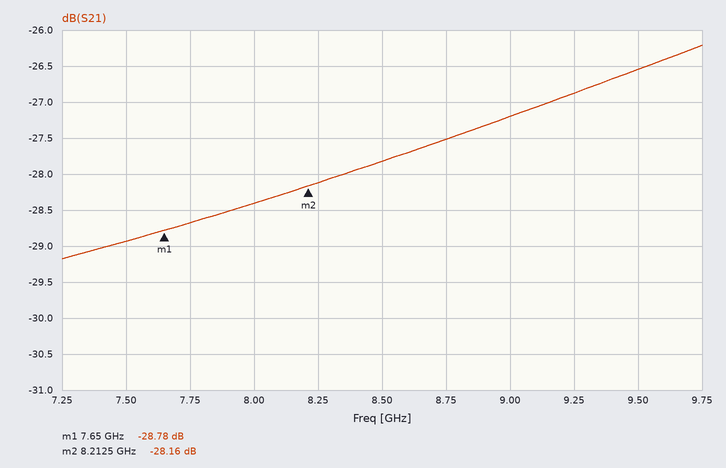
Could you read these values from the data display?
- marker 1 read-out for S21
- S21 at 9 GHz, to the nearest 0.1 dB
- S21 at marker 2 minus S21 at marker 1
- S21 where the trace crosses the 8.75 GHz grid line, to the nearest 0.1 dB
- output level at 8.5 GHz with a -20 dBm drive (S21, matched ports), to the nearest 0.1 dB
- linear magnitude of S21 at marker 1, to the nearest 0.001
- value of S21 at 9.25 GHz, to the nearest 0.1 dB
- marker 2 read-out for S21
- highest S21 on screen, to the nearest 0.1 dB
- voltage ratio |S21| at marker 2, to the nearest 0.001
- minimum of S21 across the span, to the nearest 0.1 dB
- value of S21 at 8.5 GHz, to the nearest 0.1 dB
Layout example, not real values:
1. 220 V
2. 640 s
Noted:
1. -28.78 dB
2. -27.2 dB
3. 0.62 dB
4. -27.5 dB
5. -47.8 dBm
6. 0.036
7. -26.9 dB
8. -28.16 dB
9. -26.2 dB
10. 0.039
11. -29.2 dB
12. -27.8 dB
